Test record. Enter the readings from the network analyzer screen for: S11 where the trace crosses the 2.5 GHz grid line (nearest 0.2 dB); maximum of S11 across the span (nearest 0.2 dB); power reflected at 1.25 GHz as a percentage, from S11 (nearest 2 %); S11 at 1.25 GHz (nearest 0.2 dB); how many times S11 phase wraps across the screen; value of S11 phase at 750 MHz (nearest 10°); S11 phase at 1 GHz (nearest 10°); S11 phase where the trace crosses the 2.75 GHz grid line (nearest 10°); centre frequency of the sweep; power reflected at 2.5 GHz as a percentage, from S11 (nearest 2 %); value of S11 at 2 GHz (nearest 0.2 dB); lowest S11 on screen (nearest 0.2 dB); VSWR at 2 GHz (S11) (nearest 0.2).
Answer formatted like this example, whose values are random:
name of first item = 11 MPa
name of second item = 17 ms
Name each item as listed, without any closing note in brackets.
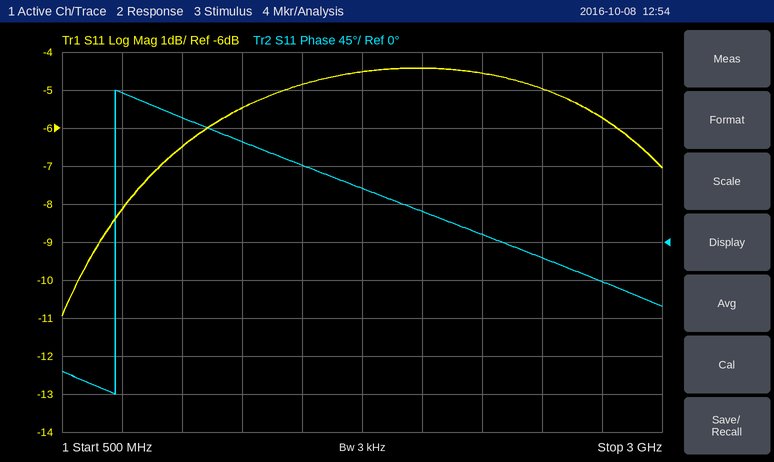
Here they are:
S11 where the trace crosses the 2.5 GHz grid line = -5.0 dB
maximum of S11 across the span = -4.4 dB
power reflected at 1.25 GHz as a percentage, from S11 = 28 %
S11 at 1.25 GHz = -5.4 dB
how many times S11 phase wraps across the screen = 1
value of S11 phase at 750 MHz = 180°
S11 phase at 1 GHz = 150°
S11 phase where the trace crosses the 2.75 GHz grid line = -50°
centre frequency of the sweep = 1.75 GHz
power reflected at 2.5 GHz as a percentage, from S11 = 32 %
value of S11 at 2 GHz = -4.4 dB
lowest S11 on screen = -11.0 dB
VSWR at 2 GHz (S11) = 4.0
